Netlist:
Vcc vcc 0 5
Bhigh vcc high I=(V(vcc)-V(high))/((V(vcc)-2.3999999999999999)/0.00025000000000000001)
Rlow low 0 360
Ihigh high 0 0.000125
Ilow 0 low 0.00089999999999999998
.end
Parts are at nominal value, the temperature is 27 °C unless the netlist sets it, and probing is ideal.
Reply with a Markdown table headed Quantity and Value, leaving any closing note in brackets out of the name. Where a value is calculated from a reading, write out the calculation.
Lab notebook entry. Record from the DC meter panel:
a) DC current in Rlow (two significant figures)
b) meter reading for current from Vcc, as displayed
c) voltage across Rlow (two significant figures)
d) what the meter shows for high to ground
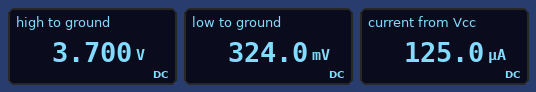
| Quantity | Value |
|---|---|
| DC current in Rlow | (324 mV) / 360 Ω = 900 µA |
| meter reading for current from Vcc, as displayed | 125.0 µA |
| voltage across Rlow | 324 mV = 320 mV |
| what the meter shows for high to ground | 3.700 V |
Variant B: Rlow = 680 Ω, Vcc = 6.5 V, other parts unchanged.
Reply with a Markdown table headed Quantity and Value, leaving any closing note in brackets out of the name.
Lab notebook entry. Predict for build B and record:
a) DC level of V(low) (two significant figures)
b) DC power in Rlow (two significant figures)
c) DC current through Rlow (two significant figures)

| Quantity | Value |
|---|---|
| DC level of V(low) | 610 mV |
| DC power in Rlow | 550 µW |
| DC current through Rlow | 900 µA |
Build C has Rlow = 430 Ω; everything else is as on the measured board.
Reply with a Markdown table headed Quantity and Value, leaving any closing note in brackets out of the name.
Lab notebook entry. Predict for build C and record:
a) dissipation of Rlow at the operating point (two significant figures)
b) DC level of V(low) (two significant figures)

| Quantity | Value |
|---|---|
| dissipation of Rlow at the operating point | 350 µW |
| DC level of V(low) | 390 mV |
